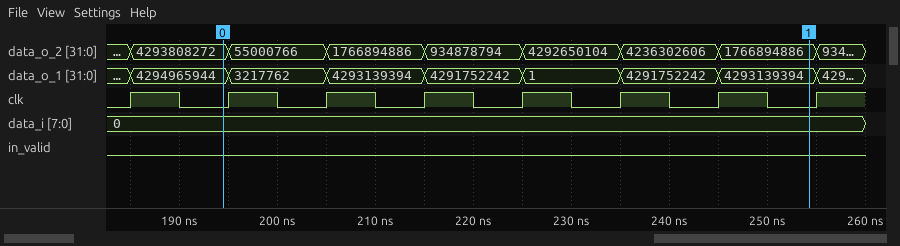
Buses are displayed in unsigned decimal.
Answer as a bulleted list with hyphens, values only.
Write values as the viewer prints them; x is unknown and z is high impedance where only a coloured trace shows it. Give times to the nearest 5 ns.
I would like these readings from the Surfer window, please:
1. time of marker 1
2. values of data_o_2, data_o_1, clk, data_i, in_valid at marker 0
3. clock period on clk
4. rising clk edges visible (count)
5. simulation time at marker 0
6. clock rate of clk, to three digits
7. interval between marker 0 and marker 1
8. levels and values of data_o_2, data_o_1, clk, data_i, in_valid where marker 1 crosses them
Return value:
- 255 ns
- data_o_2=4293808272, data_o_1=4294965944, clk=0, data_i=0, in_valid=0
- 10 ns
- 8
- 195 ns
- 100 MHz
- 60 ns
- data_o_2=1766894886, data_o_1=4293139394, clk=0, data_i=0, in_valid=0
